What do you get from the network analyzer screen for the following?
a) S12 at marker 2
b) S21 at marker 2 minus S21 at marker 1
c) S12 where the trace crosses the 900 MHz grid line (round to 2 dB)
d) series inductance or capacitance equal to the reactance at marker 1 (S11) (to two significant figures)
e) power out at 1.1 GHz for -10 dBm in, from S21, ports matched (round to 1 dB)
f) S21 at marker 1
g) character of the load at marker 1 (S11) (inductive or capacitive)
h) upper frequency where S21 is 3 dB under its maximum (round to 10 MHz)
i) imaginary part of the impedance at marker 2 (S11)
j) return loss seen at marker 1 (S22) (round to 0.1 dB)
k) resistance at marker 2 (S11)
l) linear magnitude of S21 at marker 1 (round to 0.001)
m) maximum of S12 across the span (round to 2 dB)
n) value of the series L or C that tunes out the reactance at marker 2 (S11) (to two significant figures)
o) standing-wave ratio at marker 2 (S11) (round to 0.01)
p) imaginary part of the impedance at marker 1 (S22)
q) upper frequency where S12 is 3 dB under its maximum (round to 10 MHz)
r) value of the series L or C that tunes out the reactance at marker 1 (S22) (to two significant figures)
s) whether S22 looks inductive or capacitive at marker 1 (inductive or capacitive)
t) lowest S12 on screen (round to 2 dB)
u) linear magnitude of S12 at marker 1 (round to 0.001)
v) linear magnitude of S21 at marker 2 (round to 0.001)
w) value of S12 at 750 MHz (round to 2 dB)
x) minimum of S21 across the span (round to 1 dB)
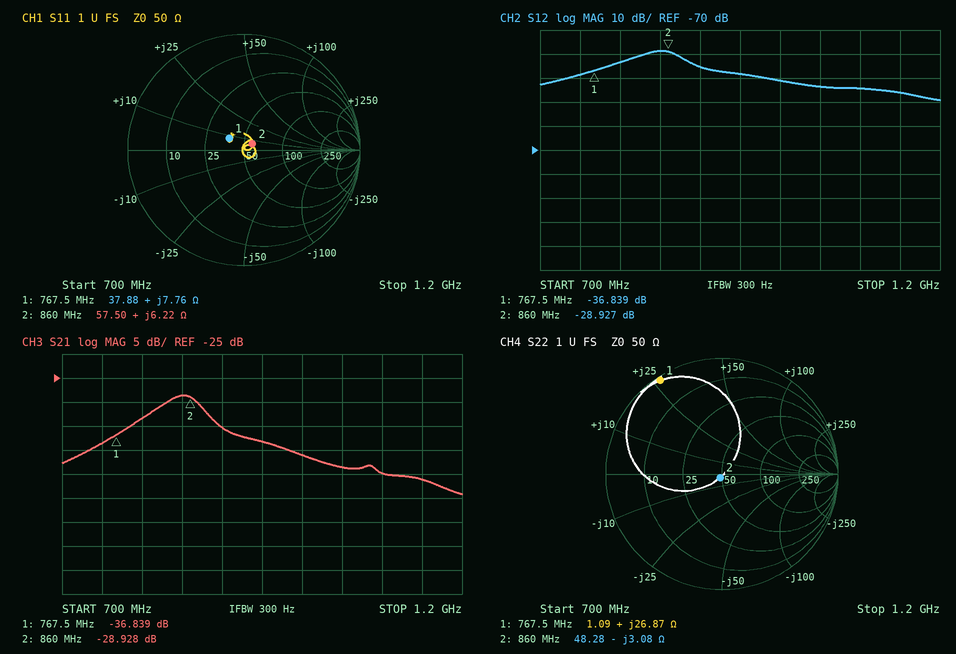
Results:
-28.927 dB
7.911 dB
-36 dB
1.6 nH
-55 dBm
-36.839 dB
inductive
880 MHz
+6.22 Ω
0.3 dB
57.50 Ω
0.014
-28 dB
30 pF
1.20
+26.87 Ω
880 MHz
7.7 pF
inductive
-50 dB
0.014
0.036
-38 dB
-49 dB
